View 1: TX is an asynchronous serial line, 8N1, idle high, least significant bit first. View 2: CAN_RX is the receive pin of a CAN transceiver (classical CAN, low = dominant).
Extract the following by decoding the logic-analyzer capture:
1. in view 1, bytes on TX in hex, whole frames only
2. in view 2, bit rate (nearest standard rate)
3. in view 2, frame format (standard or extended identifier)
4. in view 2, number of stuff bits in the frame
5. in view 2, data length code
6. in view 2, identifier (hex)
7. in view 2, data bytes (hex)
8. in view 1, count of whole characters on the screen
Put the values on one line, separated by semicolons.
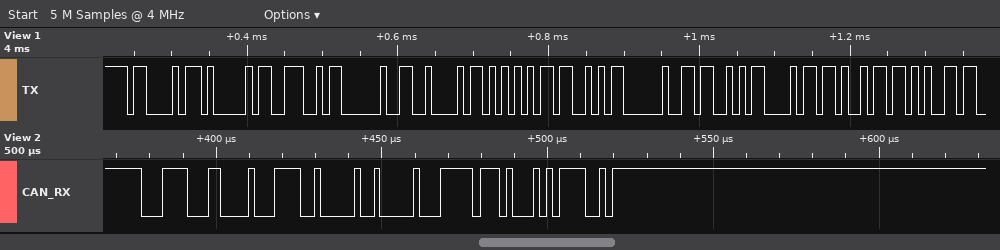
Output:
0x43 0x41 0x4E 0x20 0x42 0x55 0x53 0x20 0x53 0x68 0x69 0x65; 500 kbit/s; standard; 3; 4; 0x1E3; 79 01 00 FF; 12
